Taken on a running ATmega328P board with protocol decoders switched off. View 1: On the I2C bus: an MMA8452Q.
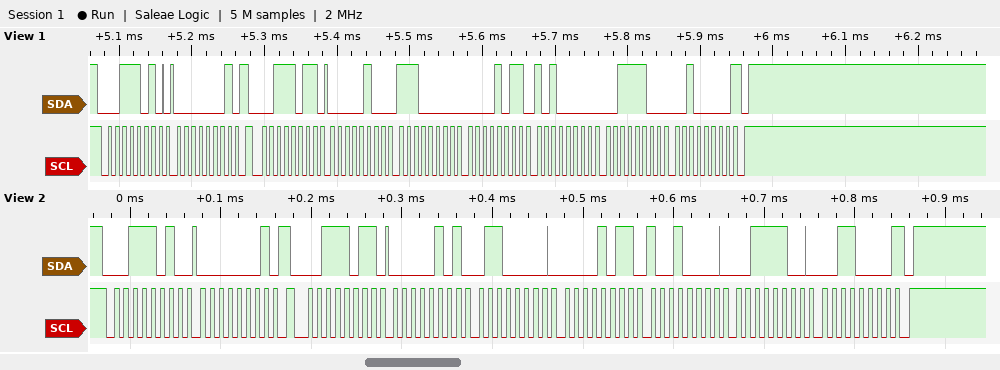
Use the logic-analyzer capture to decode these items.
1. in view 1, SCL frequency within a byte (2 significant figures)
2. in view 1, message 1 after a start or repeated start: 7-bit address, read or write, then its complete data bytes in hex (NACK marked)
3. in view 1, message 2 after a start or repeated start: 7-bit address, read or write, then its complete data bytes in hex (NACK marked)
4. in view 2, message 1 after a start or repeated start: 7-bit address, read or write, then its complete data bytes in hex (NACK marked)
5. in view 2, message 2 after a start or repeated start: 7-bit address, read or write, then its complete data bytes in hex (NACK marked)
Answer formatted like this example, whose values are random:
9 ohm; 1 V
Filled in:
100 kHz; 0x1D write: 01; 0x1D read: 04 E0 0B A0 3C 20 NACK; 0x1D write: 01; 0x1D read: 05 60 0B 90 3C 30 NACK
